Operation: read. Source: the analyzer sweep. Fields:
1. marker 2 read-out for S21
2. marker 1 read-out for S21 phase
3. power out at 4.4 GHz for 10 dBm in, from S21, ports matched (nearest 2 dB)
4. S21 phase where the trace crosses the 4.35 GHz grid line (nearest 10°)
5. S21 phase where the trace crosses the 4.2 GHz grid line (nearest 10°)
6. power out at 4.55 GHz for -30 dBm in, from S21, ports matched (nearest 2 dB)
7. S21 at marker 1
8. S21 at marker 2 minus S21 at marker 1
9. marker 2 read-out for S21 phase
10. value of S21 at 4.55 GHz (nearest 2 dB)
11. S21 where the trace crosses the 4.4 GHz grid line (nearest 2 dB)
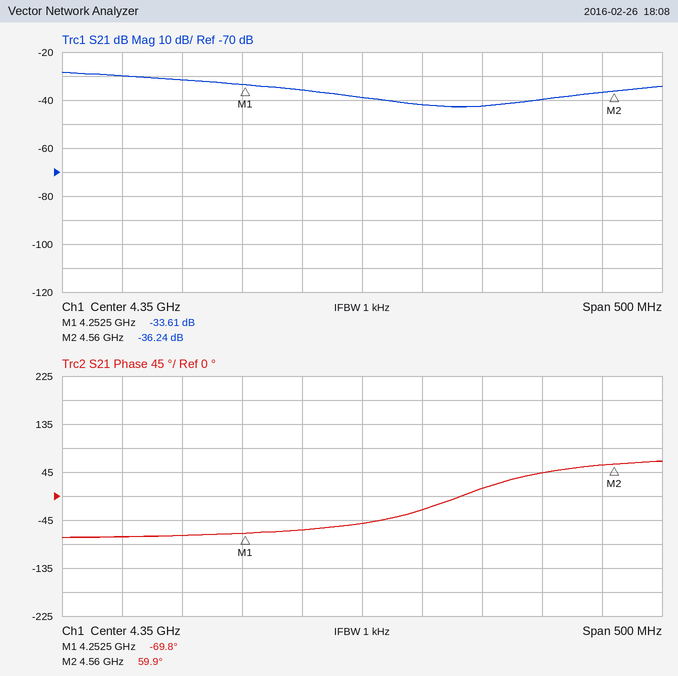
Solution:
-36.24 dB
-69.8°
-32 dBm
-50°
-70°
-66 dBm
-33.61 dB
-2.63 dB
59.9°
-36 dB
-42 dB
